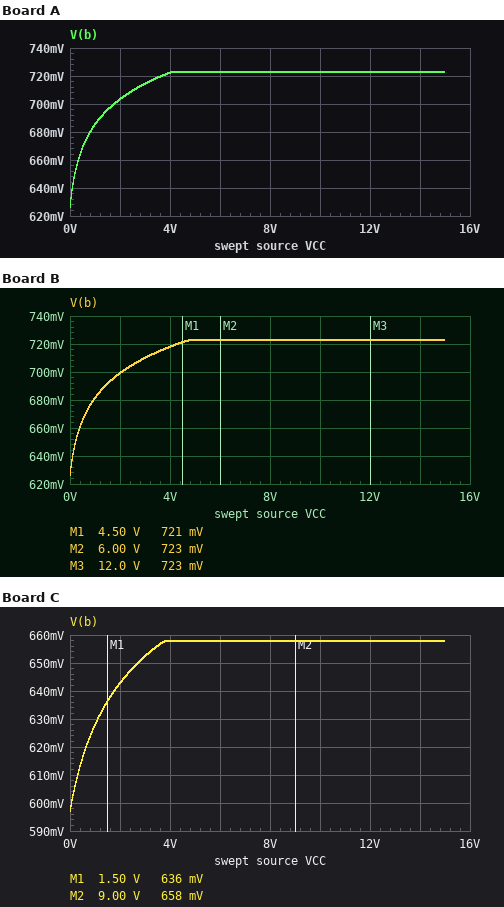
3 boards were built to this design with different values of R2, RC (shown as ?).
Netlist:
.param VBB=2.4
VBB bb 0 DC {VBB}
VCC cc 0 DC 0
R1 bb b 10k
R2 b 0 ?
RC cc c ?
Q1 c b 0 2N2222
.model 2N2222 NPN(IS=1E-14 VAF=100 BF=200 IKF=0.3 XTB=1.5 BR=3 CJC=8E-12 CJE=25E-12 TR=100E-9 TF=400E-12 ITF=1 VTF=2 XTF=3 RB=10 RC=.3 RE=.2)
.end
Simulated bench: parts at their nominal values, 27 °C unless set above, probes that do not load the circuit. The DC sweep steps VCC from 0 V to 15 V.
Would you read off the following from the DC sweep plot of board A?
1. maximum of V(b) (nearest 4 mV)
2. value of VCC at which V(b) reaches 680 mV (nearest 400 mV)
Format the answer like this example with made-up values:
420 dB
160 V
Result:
724 mV
800 mV
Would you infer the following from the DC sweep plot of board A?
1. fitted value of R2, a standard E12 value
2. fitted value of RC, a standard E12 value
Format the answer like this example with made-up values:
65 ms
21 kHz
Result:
6.8 kΩ
330 Ω
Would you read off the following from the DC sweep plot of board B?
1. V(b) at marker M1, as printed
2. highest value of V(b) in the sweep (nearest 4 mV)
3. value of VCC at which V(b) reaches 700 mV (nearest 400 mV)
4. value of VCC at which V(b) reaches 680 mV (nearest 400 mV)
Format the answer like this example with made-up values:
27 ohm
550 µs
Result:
721 mV
724 mV
2.0 V
800 mV
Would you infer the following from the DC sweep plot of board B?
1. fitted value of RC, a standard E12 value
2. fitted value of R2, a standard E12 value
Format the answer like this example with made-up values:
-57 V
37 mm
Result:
390 Ω
6.8 kΩ
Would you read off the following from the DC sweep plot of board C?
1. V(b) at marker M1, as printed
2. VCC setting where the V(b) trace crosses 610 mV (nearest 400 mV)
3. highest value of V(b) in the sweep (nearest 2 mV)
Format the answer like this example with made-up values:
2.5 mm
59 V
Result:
636 mV
400 mV
658 mV
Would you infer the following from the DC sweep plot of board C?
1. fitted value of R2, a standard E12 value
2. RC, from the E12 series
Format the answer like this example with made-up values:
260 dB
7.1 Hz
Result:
3.9 kΩ
3.3 kΩ
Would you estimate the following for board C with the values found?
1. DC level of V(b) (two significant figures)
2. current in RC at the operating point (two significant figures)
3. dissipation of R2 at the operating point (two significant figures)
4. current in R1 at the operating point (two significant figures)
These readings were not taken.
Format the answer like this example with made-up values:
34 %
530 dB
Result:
600 mV
2.1 µA
91 µW
180 µA
